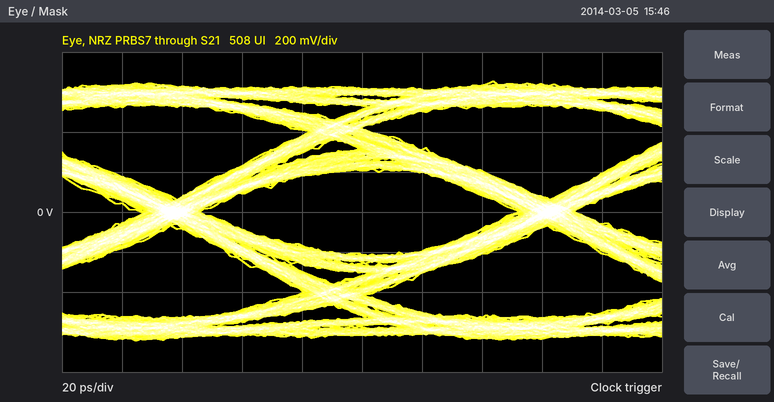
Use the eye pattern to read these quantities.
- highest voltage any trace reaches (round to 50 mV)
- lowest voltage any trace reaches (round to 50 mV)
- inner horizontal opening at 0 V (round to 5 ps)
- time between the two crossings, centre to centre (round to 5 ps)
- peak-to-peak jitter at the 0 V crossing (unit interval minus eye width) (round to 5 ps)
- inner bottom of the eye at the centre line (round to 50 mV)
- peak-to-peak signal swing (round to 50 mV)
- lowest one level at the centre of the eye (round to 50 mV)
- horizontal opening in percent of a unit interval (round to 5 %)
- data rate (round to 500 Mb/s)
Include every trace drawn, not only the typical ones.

650 mV
-650 mV
105 ps
125 ps
20 ps
-200 mV
1.30 V
200 mV
85 %
8.0 Gb/s
